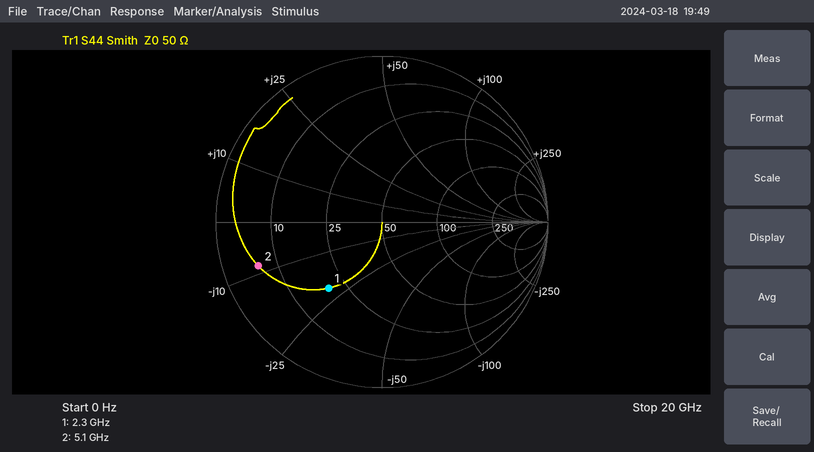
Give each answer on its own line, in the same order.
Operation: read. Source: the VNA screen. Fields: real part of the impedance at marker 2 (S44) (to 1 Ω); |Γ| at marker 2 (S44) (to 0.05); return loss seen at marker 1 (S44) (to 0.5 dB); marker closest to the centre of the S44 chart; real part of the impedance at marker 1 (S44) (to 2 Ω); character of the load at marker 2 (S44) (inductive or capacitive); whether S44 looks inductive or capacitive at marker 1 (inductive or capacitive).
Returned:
6 Ω
0.80
6.0 dB
marker 1
20 Ω
capacitive
capacitive
